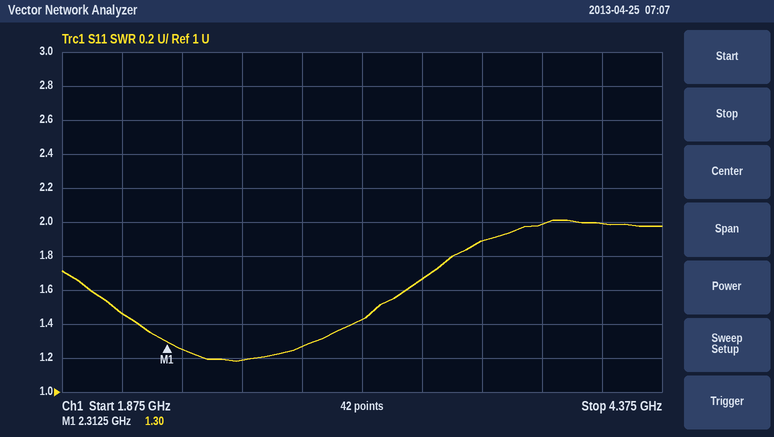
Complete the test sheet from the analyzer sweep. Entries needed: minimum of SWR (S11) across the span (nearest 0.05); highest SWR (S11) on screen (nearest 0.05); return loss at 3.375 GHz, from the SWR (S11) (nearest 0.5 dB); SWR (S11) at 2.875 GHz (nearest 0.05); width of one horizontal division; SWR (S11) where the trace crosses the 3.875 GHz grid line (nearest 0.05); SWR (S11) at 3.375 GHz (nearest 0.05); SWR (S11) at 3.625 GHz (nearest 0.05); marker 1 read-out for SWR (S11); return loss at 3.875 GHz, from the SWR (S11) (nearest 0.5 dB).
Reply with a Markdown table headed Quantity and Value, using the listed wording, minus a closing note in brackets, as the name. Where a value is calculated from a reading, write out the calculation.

| Quantity | Value |
|---|---|
| minimum of SWR (S11) across the span | 1.20 |
| highest SWR (S11) on screen | 2.00 |
| return loss at 3.375 GHz, from the SWR (S11) | −20 log10((1.65 − 1)/(1.65 + 1)) ≈ 12.2 dB, so 12.0 dB to the nearest 0.5 dB |
| SWR (S11) at 2.875 GHz | 1.25 |
| width of one horizontal division | 250 MHz |
| SWR (S11) where the trace crosses the 3.875 GHz grid line | 2.00 |
| SWR (S11) at 3.375 GHz | 1.65 |
| SWR (S11) at 3.625 GHz | 1.90 |
| marker 1 read-out for SWR | 1.30 |
| return loss at 3.875 GHz, from the SWR (S11) | −20 log10((2 − 1)/(2 + 1)) ≈ 9.5 dB |
